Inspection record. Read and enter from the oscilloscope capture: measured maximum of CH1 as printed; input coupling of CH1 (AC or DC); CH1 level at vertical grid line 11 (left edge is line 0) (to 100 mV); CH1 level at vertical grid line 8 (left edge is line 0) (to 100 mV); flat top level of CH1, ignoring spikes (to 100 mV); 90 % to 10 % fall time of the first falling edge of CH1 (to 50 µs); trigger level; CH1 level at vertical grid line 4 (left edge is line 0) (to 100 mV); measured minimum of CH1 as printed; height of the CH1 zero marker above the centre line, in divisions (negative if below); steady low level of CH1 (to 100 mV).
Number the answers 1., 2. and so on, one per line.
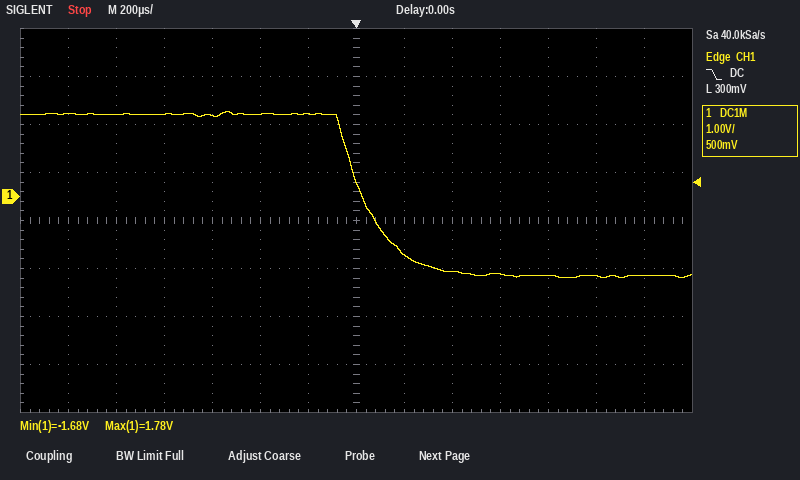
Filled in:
1. 1.78 V
2. DC
3. -1.6 V
4. -1.2 V
5. 1.7 V
6. 300 µs
7. 300 mV
8. 1.7 V
9. -1.68 V
10. +0.5 div
11. -1.6 V
